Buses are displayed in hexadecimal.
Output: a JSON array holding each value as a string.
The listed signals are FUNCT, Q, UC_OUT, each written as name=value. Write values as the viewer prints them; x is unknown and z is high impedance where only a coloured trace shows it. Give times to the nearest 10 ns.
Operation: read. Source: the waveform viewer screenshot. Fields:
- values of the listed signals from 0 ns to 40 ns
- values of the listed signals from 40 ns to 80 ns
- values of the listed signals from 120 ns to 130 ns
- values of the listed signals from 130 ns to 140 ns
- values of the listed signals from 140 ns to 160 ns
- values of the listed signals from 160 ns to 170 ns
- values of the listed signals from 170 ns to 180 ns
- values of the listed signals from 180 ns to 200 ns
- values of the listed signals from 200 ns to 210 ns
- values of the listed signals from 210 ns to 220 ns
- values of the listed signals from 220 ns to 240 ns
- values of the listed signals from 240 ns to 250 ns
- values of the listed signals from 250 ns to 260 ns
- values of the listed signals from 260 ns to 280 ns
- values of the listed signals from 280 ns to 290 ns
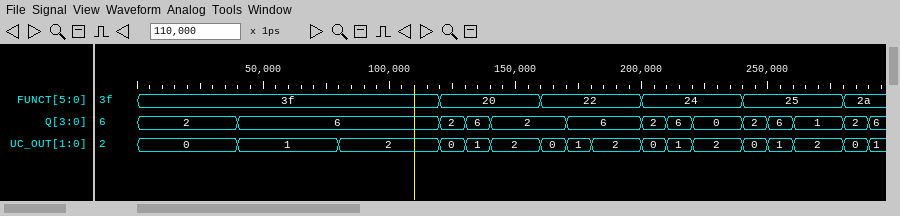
["FUNCT=3f, Q=2, UC_OUT=0", "FUNCT=3f, Q=6, UC_OUT=1", "FUNCT=20, Q=2, UC_OUT=0", "FUNCT=20, Q=6, UC_OUT=1", "FUNCT=20, Q=2, UC_OUT=2", "FUNCT=22, Q=2, UC_OUT=0", "FUNCT=22, Q=6, UC_OUT=1", "FUNCT=22, Q=6, UC_OUT=2", "FUNCT=24, Q=2, UC_OUT=0", "FUNCT=24, Q=6, UC_OUT=1", "FUNCT=24, Q=0, UC_OUT=2", "FUNCT=25, Q=2, UC_OUT=0", "FUNCT=25, Q=6, UC_OUT=1", "FUNCT=25, Q=1, UC_OUT=2", "FUNCT=2a, Q=2, UC_OUT=0"]
